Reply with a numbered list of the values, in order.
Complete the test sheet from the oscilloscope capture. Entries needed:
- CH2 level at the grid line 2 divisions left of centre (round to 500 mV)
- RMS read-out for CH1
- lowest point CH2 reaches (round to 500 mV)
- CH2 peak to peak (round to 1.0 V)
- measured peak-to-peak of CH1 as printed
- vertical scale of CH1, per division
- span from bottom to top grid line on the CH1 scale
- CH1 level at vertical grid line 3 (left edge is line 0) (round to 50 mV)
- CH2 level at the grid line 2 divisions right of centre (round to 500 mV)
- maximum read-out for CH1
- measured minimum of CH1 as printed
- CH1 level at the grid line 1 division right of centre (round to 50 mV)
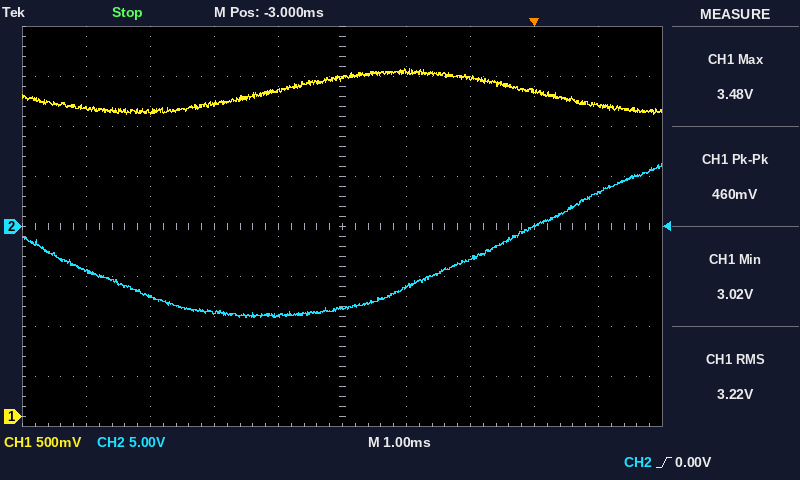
1. -8.5 V
2. 3.22 V
3. -9.0 V
4. 15.0 V
5. 460 mV
6. 500 mV
7. 4 V
8. 3.15 V
9. -3.0 V
10. 3.48 V
11. 3.02 V
12. 3.45 V
